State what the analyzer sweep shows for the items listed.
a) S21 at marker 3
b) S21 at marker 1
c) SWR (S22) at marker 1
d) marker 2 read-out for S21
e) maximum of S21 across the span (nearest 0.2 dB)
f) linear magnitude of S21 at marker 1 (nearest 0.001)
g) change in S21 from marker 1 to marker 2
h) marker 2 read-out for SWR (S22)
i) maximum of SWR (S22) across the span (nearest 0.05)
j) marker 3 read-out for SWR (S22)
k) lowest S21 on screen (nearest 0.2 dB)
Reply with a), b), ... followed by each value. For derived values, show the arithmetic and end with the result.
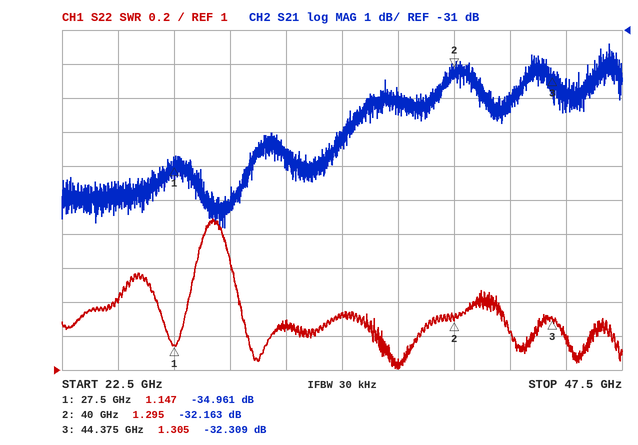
a) -32.309 dB
b) -34.961 dB
c) 1.147
d) -32.163 dB
e) -31.4 dB
f) 10^(-34.961/20) ≈ 0.018
g) -32.163 − (-34.961) = 2.798 dB
h) 1.295
i) 1.90
j) 1.305
k) -36.8 dB
